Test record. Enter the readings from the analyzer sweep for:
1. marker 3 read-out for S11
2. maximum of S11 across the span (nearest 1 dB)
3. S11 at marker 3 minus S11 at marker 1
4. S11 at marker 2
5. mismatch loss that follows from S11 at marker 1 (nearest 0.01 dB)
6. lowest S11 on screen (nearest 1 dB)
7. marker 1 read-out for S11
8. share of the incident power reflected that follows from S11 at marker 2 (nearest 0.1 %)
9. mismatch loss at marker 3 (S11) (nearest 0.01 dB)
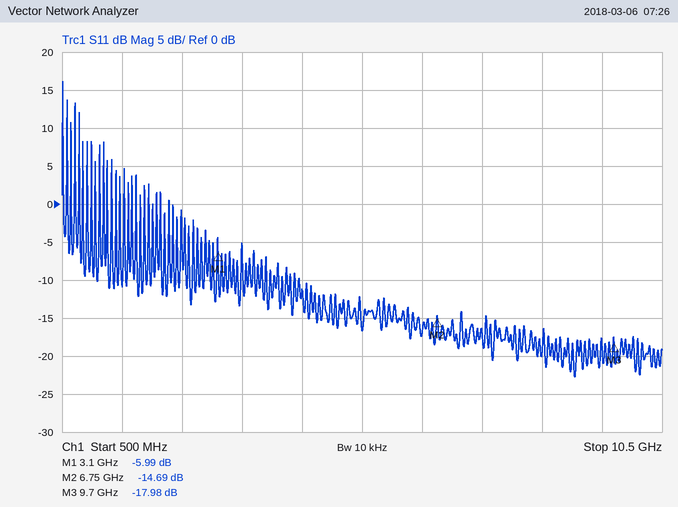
-17.98 dB
16 dB
-11.99 dB
-14.69 dB
1.26 dB
-23 dB
-5.99 dB
3.4 %
0.07 dB
